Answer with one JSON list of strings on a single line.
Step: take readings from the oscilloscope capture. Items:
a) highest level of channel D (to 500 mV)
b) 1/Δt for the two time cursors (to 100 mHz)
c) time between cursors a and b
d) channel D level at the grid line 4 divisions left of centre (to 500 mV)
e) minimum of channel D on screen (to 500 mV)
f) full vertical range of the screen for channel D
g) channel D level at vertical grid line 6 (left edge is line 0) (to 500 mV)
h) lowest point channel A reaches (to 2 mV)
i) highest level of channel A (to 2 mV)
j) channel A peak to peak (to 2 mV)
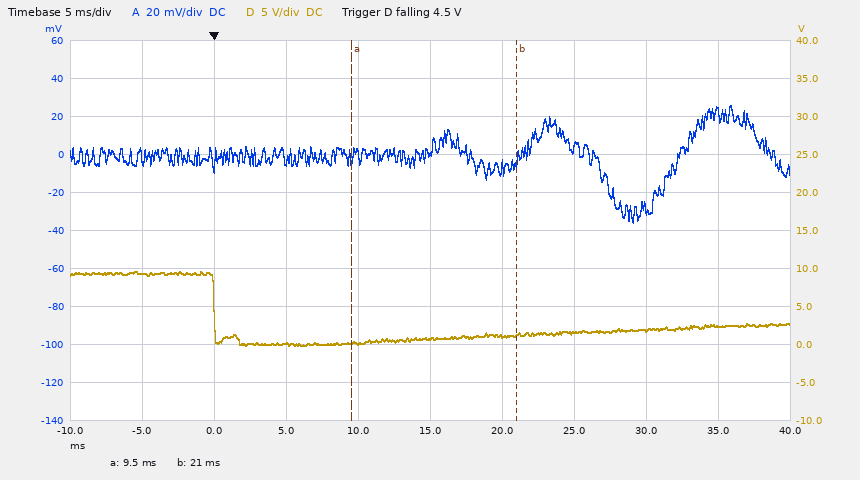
["9.5 V", "87.0 Hz", "11.5 ms", "9.5 V", "0.0 V", "50 V", "1.0 V", "-36 mV", "26 mV", "62 mV"]
